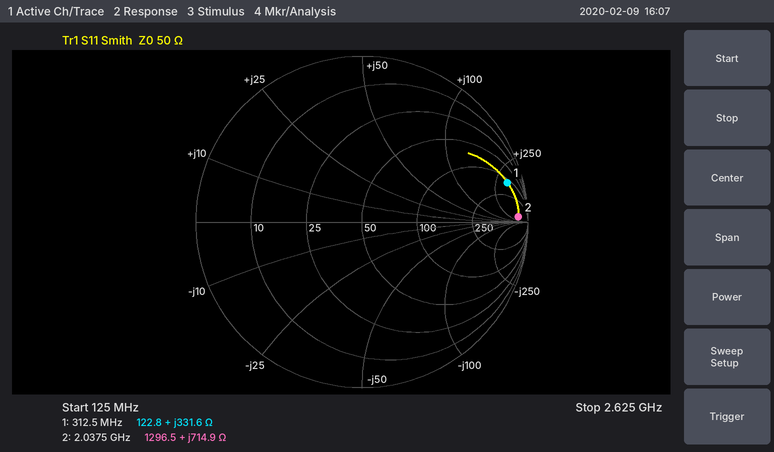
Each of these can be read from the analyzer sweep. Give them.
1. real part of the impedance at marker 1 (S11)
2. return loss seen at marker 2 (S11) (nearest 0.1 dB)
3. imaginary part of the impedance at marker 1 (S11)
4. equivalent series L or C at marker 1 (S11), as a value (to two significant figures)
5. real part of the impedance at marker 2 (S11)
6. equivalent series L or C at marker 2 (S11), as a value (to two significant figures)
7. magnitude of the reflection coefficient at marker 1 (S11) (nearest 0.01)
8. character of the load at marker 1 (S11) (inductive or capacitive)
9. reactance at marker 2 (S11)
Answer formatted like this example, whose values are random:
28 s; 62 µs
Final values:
122.8 Ω; 0.5 dB; +331.6 Ω; 170 nH; 1296.5 Ω; 56 nH; 0.91; inductive; +714.9 Ω
